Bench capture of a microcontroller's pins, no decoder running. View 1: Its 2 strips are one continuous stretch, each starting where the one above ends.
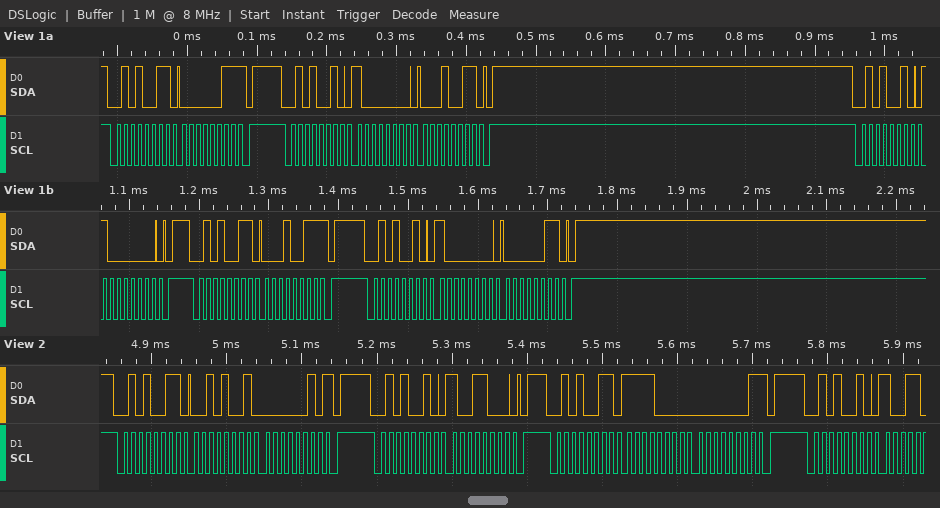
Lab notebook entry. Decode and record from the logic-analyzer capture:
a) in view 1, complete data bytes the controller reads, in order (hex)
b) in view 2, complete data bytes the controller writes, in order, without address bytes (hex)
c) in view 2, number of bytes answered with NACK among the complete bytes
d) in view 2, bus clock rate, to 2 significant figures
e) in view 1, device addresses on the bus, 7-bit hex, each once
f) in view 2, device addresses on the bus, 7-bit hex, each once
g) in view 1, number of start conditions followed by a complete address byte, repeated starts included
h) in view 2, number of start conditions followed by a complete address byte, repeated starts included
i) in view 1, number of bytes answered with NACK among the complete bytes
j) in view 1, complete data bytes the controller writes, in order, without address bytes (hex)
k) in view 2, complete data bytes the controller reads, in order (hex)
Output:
03 13
98
2
100 kHz
0x29
0x29
5
4
2
80 13 80 80 03
29 02 F0 01
